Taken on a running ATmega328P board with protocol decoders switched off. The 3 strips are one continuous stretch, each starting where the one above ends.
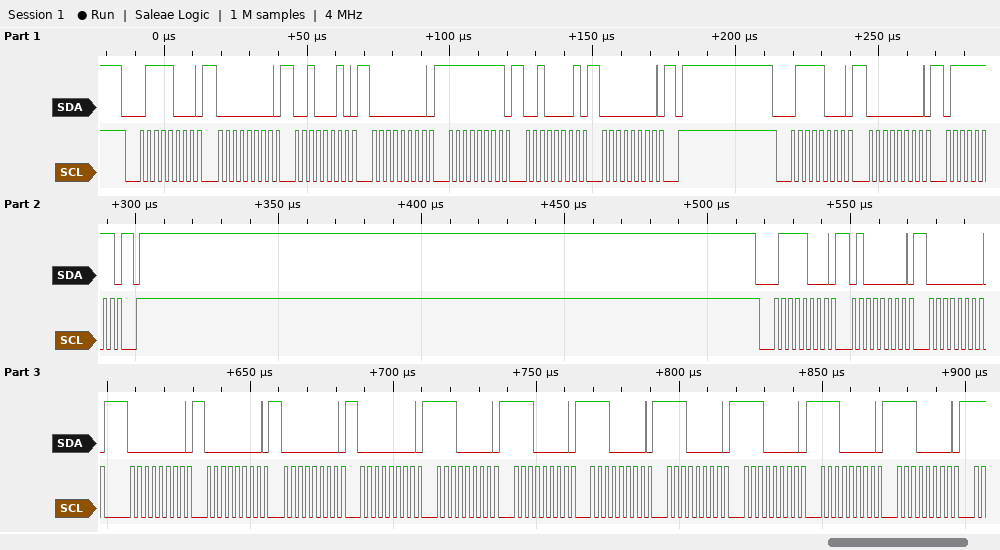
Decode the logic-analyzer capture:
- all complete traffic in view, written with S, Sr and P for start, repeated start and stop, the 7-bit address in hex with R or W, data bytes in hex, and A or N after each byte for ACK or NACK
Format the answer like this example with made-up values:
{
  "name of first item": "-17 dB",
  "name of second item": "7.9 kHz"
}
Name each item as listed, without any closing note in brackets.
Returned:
{
  "all complete traffic in view, written with S, Sr and P for start, repeated start and stop, the 7-bit address in hex with R or W, data bytes in hex, and A or N after each byte for ACK or NACK": "S 3CW A 00 A 22 A 00 A FF A 21 A 00 A P S 3CW A 00 A 7F A P S 3CW A 40 A 00 A 00 A 00 A 00 A 00 A E0 A E0 A E0 A E0 A E0 A E0 A E0 A"
}
